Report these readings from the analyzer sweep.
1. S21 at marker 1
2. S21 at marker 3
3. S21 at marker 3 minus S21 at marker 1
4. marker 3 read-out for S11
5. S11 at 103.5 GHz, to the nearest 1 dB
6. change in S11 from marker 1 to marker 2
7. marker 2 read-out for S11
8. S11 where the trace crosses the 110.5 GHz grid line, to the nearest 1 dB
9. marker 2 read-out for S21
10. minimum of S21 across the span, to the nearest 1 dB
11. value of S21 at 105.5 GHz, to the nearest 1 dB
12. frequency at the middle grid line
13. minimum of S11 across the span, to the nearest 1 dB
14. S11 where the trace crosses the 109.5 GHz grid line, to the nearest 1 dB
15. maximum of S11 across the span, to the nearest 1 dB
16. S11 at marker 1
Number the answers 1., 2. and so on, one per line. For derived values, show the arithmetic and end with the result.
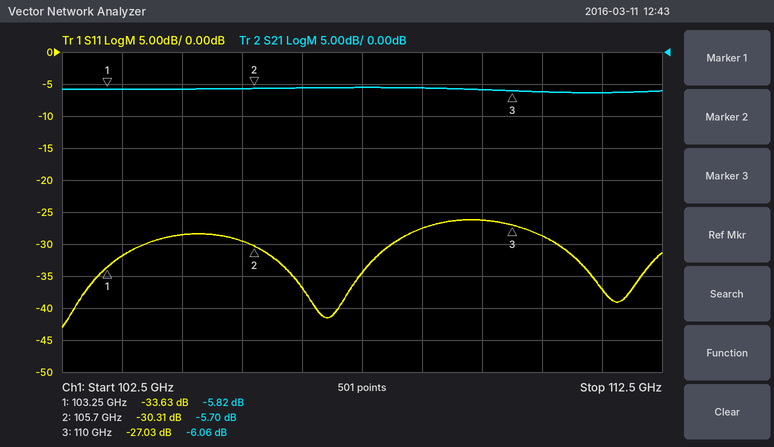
1. -5.82 dB
2. -6.06 dB
3. -6.06 − (-5.82) = -0.24 dB
4. -27.03 dB
5. -32 dB
6. -30.31 − (-33.63) = 3.32 dB
7. -30.31 dB
8. -29 dB
9. -5.70 dB
10. -6 dB
11. -6 dB
12. 107.5 GHz
13. -43 dB
14. -26 dB
15. -26 dB
16. -33.63 dB
